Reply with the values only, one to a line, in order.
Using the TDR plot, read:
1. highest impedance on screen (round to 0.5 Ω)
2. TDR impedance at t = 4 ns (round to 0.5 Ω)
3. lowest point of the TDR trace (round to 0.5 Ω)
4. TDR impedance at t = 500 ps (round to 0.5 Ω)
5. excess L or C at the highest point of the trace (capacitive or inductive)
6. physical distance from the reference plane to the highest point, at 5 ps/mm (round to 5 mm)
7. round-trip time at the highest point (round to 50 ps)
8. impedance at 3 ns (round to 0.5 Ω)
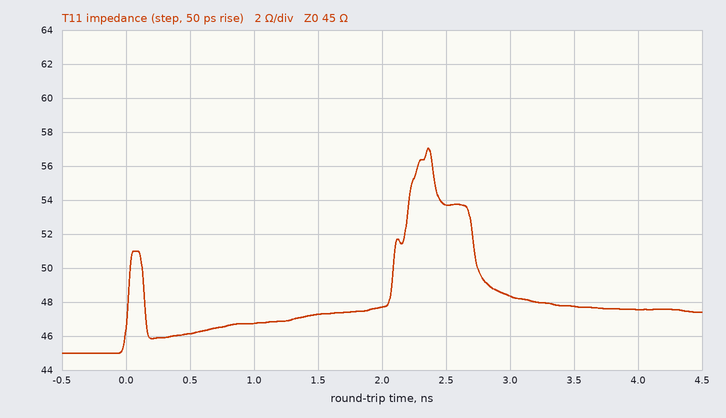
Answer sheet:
57.0 Ω
47.5 Ω
45.0 Ω
46.0 Ω
inductive
235 mm
2.35 ns
48.5 Ω
